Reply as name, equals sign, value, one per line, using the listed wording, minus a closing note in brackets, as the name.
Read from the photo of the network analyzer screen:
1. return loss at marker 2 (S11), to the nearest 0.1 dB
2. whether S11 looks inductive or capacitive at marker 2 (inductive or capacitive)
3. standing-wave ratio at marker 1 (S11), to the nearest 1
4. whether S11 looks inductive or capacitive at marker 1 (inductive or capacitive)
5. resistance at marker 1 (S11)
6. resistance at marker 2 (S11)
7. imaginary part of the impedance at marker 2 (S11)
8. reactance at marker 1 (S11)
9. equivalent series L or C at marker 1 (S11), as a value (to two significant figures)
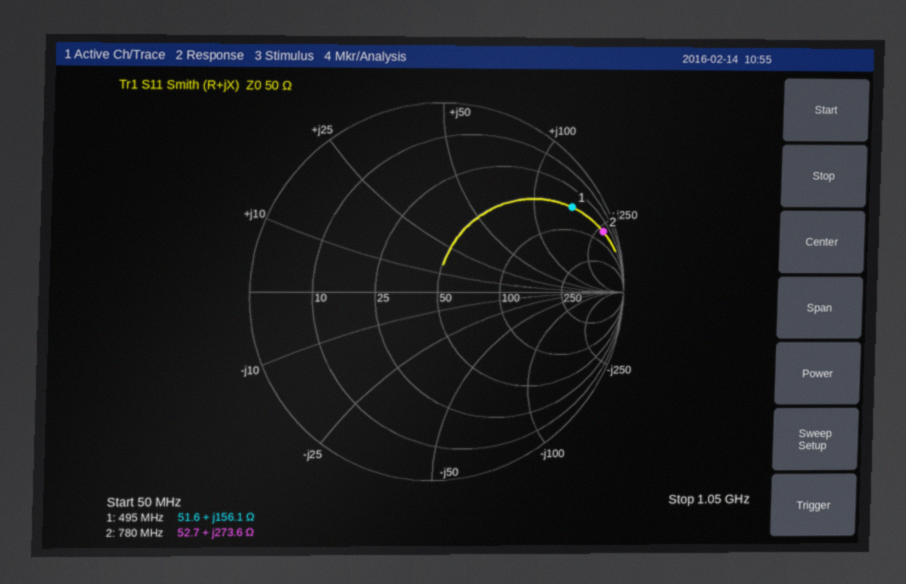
return loss at marker 2 (S11), to the nearest 0.1 dB = 0.6 dB
whether S11 looks inductive or capacitive at marker 2 = inductive
standing-wave ratio at marker 1 (S11), to the nearest 1 = 11
whether S11 looks inductive or capacitive at marker 1 = inductive
resistance at marker 1 = 51.6 Ω
resistance at marker 2 = 52.7 Ω
imaginary part of the impedance at marker 2 = +273.6 Ω
reactance at marker 1 = +156.1 Ω
equivalent series L or C at marker 1 (S11), as a value = 50 nH
